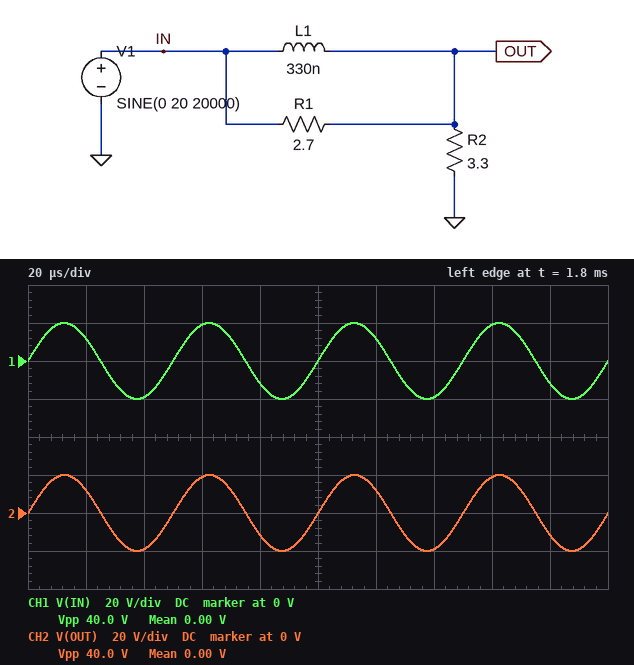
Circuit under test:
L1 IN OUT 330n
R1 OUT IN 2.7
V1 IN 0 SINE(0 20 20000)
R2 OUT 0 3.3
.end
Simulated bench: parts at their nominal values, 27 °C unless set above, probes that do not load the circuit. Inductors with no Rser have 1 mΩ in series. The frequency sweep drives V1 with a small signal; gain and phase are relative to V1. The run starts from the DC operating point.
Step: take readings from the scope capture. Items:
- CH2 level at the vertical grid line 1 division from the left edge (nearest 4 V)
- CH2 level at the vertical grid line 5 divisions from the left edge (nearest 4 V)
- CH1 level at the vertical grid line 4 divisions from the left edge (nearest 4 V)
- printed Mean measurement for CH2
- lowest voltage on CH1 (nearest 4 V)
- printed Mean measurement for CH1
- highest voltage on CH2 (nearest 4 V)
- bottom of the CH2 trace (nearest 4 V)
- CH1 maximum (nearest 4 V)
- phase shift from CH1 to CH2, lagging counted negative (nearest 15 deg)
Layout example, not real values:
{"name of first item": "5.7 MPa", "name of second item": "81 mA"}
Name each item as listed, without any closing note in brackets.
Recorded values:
{"CH2 level at the vertical grid line 1 division from the left edge": "12 V", "CH2 level at the vertical grid line 5 divisions from the left edge": "0 V", "CH1 level at the vertical grid line 4 divisions from the left edge": "-12 V", "printed Mean measurement for CH2": "0.00 V", "lowest voltage on CH1": "-20 V", "printed Mean measurement for CH1": "0.00 V", "highest voltage on CH2": "20 V", "bottom of the CH2 trace": "-20 V", "CH1 maximum": "20 V", "phase shift from CH1 to CH2, lagging counted negative": "0 deg"}
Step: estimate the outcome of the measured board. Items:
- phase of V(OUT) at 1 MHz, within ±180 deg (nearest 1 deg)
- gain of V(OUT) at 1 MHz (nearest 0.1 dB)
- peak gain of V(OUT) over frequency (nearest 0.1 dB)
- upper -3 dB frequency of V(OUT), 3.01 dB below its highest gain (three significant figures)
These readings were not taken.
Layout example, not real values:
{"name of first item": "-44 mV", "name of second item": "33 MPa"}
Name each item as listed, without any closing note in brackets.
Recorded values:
{"phase of V(OUT) at 1 MHz, within ±180 deg": "-17 deg", "gain of V(OUT) at 1 MHz": "-2.7 dB", "peak gain of V(OUT) over frequency": "0 dB", "upper -3 dB frequency of V(OUT), 3.01 dB below its highest gain": "1.14 MHz"}
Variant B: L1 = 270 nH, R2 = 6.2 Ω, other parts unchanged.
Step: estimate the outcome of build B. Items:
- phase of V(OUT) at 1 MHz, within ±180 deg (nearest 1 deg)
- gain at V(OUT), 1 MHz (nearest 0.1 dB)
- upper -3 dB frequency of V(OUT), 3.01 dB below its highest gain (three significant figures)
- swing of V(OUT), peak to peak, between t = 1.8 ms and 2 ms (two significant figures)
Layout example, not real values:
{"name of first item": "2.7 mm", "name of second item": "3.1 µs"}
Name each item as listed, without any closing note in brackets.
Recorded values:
{"phase of V(OUT) at 1 MHz, within ±180 deg": "-10 deg", "gain at V(OUT), 1 MHz": "-1.1 dB", "upper -3 dB frequency of V(OUT), 3.01 dB below its highest gain": "6.50 MHz", "swing of V(OUT), peak to peak, between t = 1.8 ms and 2 ms": "40 V"}
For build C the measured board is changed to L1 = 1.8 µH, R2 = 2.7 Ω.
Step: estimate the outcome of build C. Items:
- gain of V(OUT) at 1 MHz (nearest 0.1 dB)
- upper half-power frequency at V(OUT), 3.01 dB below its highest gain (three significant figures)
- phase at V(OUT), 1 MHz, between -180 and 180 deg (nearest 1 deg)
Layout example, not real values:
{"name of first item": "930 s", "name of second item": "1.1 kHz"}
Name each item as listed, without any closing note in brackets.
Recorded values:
{"gain of V(OUT) at 1 MHz": "-5.8 dB", "upper half-power frequency at V(OUT), 3.01 dB below its highest gain": "169 kHz", "phase at V(OUT), 1 MHz, between -180 and 180 deg": "-7 deg"}
